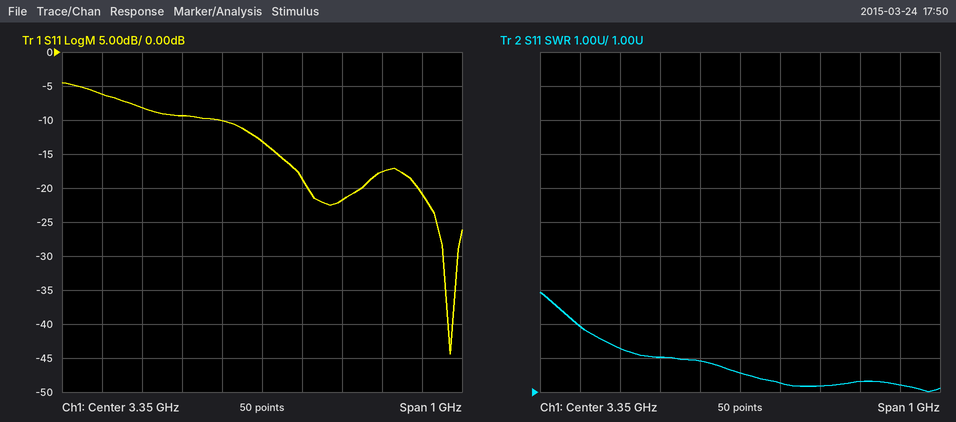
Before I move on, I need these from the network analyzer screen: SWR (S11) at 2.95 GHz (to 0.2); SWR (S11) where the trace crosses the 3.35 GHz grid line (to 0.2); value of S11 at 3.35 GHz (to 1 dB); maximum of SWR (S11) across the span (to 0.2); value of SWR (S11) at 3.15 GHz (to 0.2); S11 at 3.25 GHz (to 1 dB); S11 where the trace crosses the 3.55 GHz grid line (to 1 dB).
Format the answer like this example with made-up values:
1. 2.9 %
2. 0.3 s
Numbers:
1. 3.0
2. 1.6
3. -13 dB
4. 4.0
5. 2.0
6. -10 dB
7. -22 dB
